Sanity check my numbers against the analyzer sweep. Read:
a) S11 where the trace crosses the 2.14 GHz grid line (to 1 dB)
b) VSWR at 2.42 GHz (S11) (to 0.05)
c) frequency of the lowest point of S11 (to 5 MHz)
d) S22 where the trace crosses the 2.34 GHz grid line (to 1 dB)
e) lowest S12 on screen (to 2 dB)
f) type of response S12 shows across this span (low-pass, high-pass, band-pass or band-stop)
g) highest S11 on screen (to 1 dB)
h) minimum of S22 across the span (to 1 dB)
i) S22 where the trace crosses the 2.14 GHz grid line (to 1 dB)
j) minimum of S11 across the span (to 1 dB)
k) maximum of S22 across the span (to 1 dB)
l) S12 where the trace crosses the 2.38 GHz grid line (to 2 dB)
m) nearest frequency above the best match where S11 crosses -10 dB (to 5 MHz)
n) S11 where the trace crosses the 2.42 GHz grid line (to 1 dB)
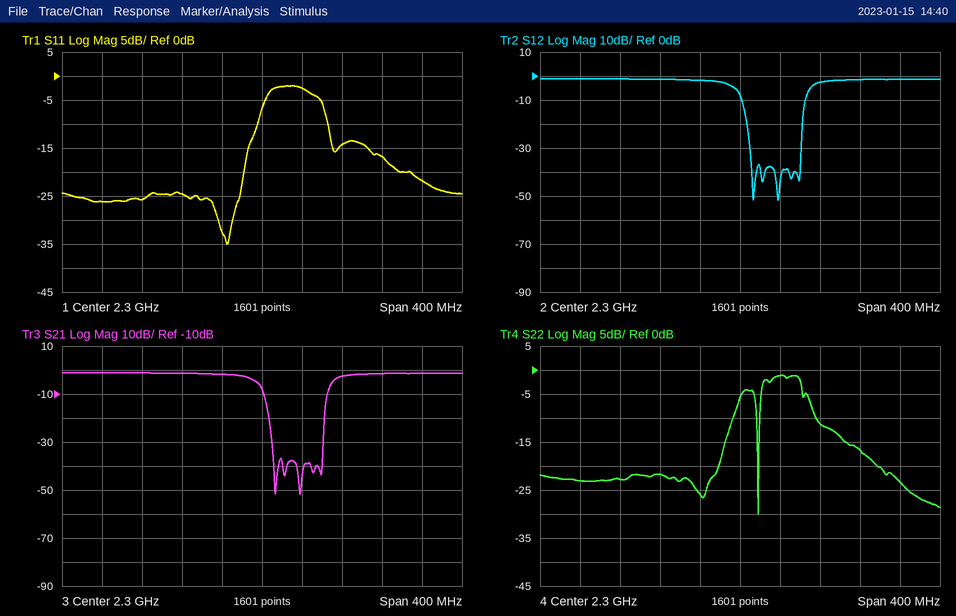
-26 dB
1.35
2.265 GHz
-1 dB
-52 dB
band-stop
-2 dB
-30 dB
-23 dB
-35 dB
-1 dB
-2 dB
2.295 GHz
-17 dB
